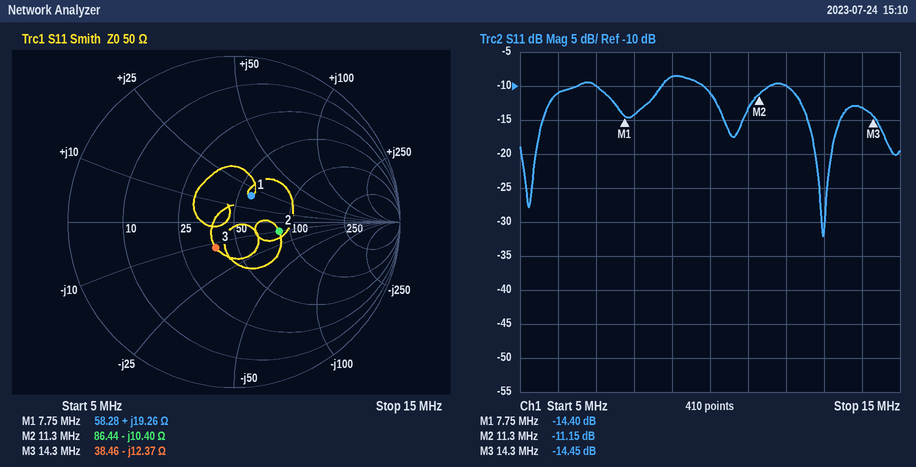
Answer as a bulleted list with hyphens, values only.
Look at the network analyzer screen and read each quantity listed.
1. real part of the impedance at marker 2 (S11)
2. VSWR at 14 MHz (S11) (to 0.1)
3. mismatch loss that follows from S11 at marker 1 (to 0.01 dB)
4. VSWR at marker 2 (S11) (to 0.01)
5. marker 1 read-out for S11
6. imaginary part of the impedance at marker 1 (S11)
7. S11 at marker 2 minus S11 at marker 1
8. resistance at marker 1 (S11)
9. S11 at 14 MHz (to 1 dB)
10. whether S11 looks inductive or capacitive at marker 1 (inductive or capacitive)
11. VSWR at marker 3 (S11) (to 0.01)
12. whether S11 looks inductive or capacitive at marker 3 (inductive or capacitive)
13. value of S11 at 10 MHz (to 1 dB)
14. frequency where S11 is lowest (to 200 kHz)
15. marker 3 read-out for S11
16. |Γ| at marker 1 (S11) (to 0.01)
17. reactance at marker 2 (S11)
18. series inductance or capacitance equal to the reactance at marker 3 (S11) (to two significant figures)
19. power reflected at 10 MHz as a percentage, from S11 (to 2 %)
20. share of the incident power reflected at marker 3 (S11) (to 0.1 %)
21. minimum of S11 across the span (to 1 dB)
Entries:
- 86.44 Ω
- 1.6
- 0.16 dB
- 1.77
- -14.40 dB
- +19.26 Ω
- 3.25 dB
- 58.28 Ω
- -13 dB
- inductive
- 1.47
- capacitive
- -11 dB
- 13.0 MHz
- -14.45 dB
- 0.19
- -10.40 Ω
- 900 pF
- 8 %
- 3.6 %
- -32 dB
